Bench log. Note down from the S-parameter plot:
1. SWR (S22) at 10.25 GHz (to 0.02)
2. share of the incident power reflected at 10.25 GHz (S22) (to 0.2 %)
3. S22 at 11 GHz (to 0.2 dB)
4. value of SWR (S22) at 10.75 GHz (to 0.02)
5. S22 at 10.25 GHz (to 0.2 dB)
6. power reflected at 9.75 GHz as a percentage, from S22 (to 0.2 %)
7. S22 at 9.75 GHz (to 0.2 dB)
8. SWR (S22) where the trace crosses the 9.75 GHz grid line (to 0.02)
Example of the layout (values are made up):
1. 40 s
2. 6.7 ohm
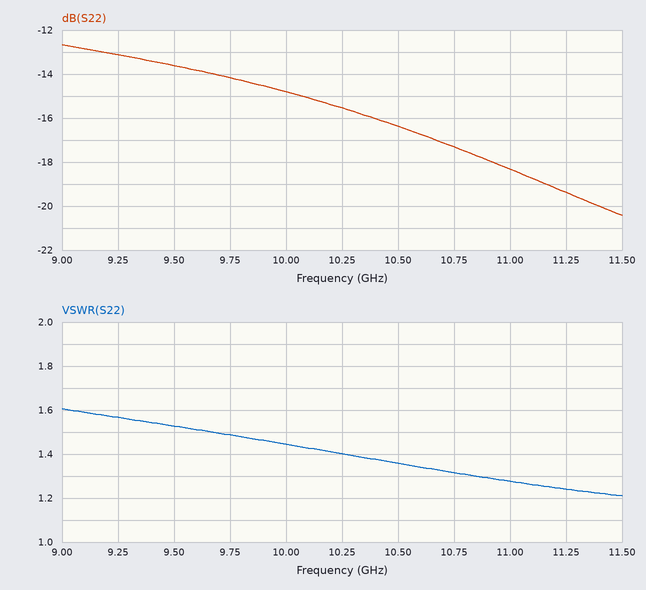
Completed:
1. 1.40
2. 2.8 %
3. -18.4 dB
4. 1.32
5. -15.6 dB
6. 3.8 %
7. -14.2 dB
8. 1.48
